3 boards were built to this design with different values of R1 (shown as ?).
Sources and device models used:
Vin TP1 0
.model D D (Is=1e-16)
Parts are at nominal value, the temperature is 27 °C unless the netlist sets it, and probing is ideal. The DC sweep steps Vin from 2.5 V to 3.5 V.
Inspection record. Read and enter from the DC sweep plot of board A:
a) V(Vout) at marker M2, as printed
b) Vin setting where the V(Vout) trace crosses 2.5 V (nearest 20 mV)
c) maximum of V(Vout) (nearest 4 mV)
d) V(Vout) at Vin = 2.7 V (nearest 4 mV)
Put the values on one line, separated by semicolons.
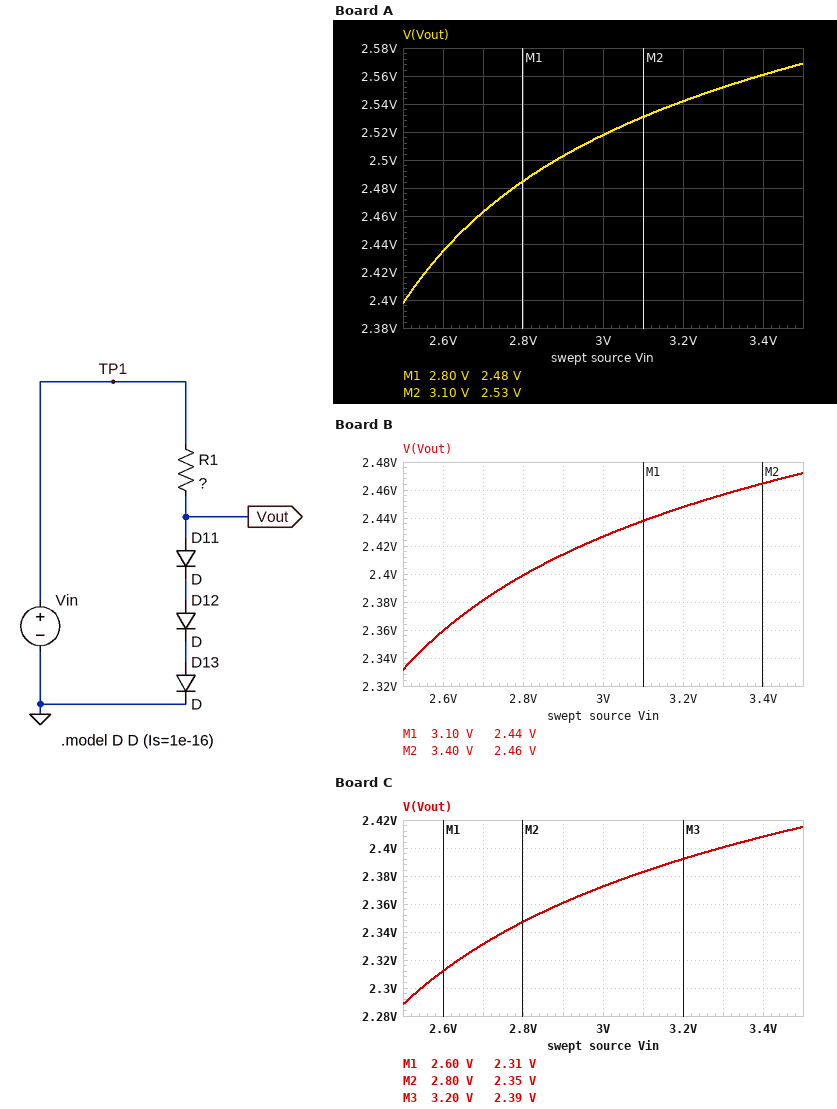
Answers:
2.53 V; 2.88 V; 2.568 V; 2.464 V
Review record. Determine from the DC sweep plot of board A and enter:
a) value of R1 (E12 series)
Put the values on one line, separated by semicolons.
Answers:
39 Ω
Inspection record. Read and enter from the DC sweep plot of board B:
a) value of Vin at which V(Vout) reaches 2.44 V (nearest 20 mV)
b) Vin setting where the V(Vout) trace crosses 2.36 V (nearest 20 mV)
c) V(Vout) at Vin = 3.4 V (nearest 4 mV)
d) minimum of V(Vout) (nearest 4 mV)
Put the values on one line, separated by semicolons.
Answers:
3.12 V; 2.60 V; 2.464 V; 2.332 V
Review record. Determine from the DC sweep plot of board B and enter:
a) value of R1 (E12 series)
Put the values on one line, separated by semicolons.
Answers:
150 Ω
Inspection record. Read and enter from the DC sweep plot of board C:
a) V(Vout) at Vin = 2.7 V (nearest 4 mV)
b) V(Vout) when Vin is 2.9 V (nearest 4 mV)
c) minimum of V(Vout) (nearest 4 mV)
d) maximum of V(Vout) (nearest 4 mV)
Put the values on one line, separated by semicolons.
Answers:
2.332 V; 2.360 V; 2.288 V; 2.416 V
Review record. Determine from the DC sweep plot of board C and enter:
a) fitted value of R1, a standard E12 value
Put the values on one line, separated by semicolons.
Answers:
330 Ω
